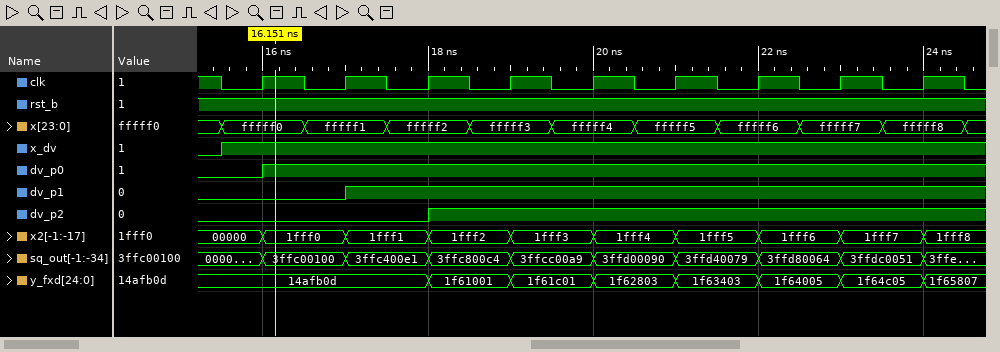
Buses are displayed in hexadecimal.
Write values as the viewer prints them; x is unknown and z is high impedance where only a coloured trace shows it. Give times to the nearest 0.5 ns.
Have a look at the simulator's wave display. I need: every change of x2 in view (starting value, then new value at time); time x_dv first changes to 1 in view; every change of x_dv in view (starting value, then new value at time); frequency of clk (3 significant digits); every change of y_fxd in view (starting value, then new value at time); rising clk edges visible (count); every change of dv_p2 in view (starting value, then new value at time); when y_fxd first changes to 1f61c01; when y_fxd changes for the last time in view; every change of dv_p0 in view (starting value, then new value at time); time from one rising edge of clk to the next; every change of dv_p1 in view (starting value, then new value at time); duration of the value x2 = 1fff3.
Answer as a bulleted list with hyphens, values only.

- 00000, 1fff0 at 16 ns, 1fff1 at 17 ns, 1fff2 at 18 ns, 1fff3 at 19 ns, 1fff4 at 20 ns, 1fff5 at 21 ns, 1fff6 at 22 ns, 1fff7 at 23 ns, 1fff8 at 24 ns
- 15.5 ns
- 0, 1 at 15.5 ns
- 1.00 GHz
- 14afb0d, 1f61001 at 18 ns, 1f61c01 at 19 ns, 1f62803 at 20 ns, 1f63403 at 21 ns, 1f64005 at 22 ns, 1f64c05 at 23 ns, 1f65807 at 24 ns
- 9
- 0, 1 at 18 ns
- 19 ns
- 24 ns
- 0, 1 at 16 ns
- 1 ns
- 0, 1 at 17 ns
- 1 ns
